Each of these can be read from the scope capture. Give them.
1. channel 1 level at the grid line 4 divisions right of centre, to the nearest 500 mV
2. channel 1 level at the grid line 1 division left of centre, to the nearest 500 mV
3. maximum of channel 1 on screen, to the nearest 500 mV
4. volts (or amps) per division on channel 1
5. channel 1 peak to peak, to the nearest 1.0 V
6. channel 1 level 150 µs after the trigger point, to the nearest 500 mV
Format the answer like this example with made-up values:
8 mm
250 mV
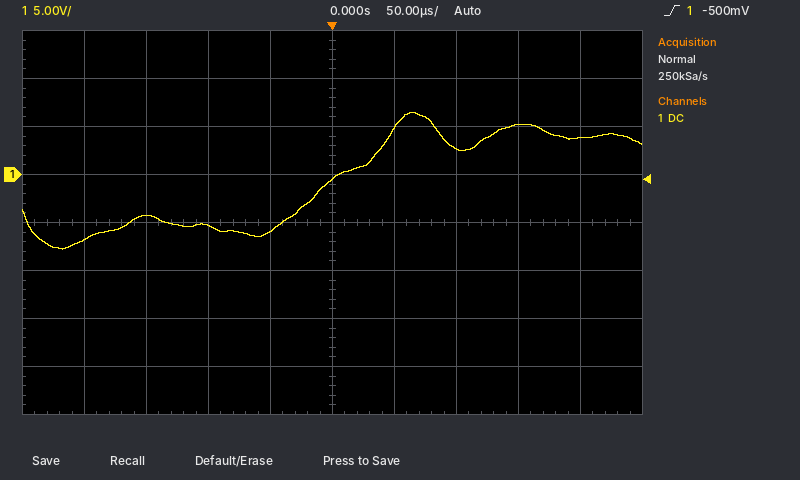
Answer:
4.0 V
-6.0 V
6.5 V
5 V
14.0 V
5.0 V
